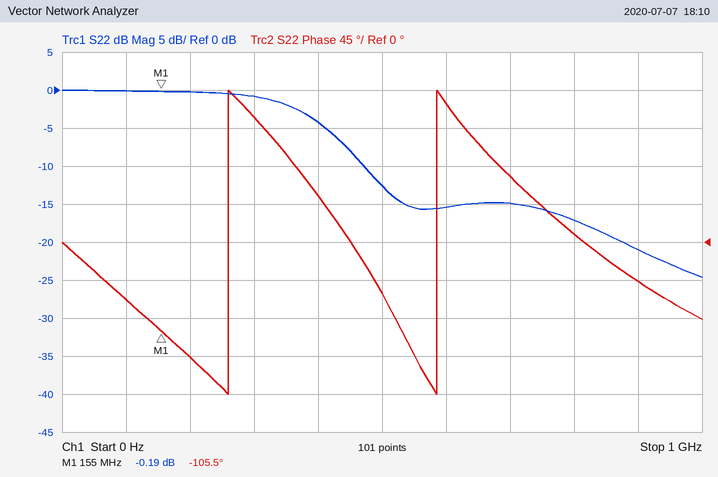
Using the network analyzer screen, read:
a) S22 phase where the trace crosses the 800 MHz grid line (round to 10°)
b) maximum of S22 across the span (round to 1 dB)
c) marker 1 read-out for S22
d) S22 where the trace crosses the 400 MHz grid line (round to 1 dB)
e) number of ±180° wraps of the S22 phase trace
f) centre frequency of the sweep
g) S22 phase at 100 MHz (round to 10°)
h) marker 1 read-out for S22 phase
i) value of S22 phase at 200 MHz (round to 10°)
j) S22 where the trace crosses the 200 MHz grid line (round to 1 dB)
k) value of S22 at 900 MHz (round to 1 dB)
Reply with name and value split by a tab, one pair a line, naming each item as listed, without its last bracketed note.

S22 phase where the trace crosses the 800 MHz grid line	10°
maximum of S22 across the span	0 dB
marker 1 read-out for S22	-0.19 dB
S22 where the trace crosses the 400 MHz grid line	-4 dB
number of ±180° wraps of the S22 phase trace	2
centre frequency of the sweep	500 MHz
S22 phase at 100 MHz	-70°
marker 1 read-out for S22 phase	-105.5°
value of S22 phase at 200 MHz	-140°
S22 where the trace crosses the 200 MHz grid line	0 dB
value of S22 at 900 MHz	-21 dB
